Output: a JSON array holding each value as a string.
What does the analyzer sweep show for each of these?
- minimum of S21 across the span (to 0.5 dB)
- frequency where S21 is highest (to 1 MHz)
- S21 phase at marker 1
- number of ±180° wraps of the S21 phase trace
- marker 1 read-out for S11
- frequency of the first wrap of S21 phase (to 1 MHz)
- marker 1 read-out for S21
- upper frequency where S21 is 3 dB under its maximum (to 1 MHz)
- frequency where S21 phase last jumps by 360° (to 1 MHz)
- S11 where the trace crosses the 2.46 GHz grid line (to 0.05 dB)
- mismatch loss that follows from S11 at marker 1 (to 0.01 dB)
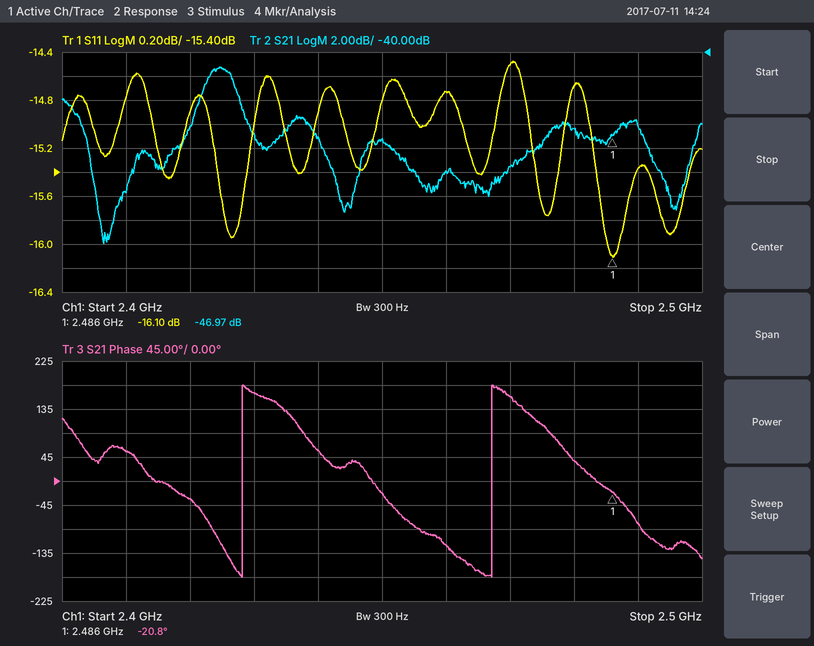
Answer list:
["-56.0 dB", "2.425 GHz", "-20.8°", "2", "-16.10 dB", "2.428 GHz", "-46.97 dB", "2.428 GHz", "2.467 GHz", "-14.75 dB", "0.11 dB"]
